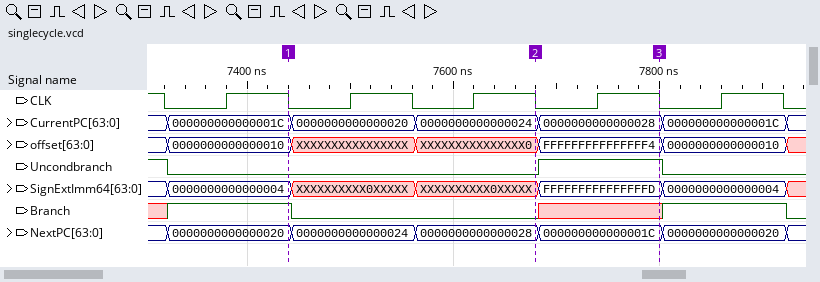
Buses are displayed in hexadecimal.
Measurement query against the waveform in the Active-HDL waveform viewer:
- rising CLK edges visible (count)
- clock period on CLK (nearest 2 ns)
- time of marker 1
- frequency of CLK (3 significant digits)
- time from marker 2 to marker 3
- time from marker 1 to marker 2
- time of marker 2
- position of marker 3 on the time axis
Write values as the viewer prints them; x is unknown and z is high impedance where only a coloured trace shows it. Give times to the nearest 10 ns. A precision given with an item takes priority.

5
120 ns
7440 ns
8.33 MHz
120 ns
240 ns
7680 ns
7800 ns
